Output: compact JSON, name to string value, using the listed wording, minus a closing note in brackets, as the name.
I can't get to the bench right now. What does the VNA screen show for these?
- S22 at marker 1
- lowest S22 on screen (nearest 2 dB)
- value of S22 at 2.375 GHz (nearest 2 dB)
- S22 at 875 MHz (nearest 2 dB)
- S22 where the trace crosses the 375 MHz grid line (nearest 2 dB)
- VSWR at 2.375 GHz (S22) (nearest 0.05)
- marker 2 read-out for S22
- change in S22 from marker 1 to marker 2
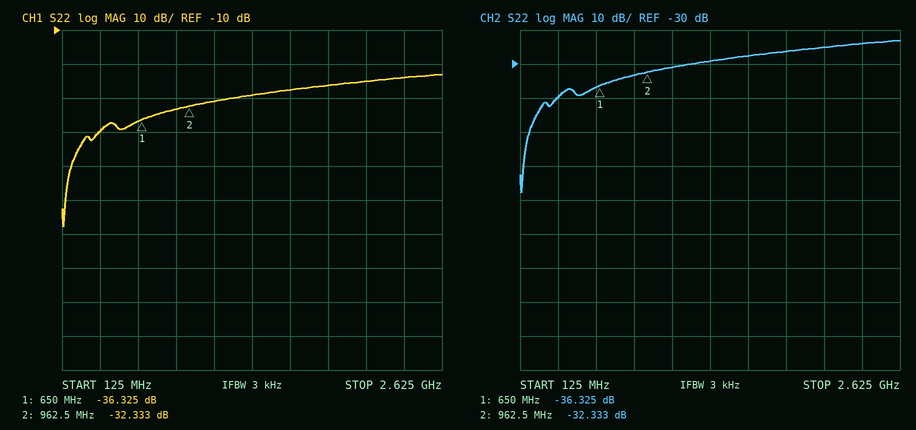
{"S22 at marker 1": "-36.325 dB", "lowest S22 on screen": "-68 dB", "value of S22 at 2.375 GHz": "-24 dB", "S22 at 875 MHz": "-34 dB", "S22 where the trace crosses the 375 MHz grid line": "-40 dB", "VSWR at 2.375 GHz (S22)": "1.15", "marker 2 read-out for S22": "-32.333 dB", "change in S22 from marker 1 to marker 2": "3.992 dB"}
